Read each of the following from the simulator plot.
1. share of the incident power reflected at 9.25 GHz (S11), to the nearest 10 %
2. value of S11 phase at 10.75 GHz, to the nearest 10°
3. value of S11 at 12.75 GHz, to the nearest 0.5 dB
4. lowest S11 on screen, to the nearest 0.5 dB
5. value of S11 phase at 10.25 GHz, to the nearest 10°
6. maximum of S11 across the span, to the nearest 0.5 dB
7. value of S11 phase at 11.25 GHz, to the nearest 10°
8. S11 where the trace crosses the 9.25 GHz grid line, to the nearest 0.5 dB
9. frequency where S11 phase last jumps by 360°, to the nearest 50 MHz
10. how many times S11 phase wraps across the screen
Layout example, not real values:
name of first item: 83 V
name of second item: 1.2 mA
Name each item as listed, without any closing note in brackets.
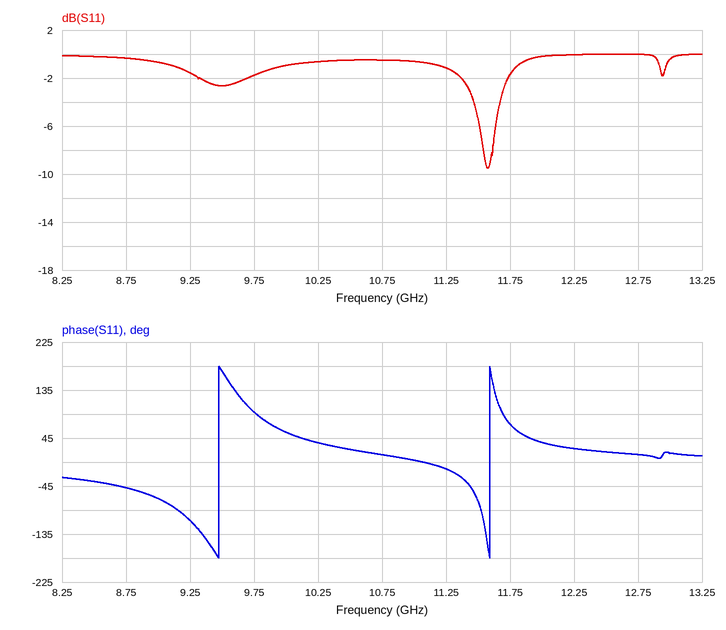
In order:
share of the incident power reflected at 9.25 GHz (S11), to the nearest 10 %: 70 %
value of S11 phase at 10.75 GHz, to the nearest 10°: 10°
value of S11 at 12.75 GHz, to the nearest 0.5 dB: 0.0 dB
lowest S11 on screen, to the nearest 0.5 dB: -9.5 dB
value of S11 phase at 10.25 GHz, to the nearest 10°: 40°
maximum of S11 across the span, to the nearest 0.5 dB: 0.0 dB
value of S11 phase at 11.25 GHz, to the nearest 10°: -10°
S11 where the trace crosses the 9.25 GHz grid line, to the nearest 0.5 dB: -1.5 dB
frequency where S11 phase last jumps by 360°, to the nearest 50 MHz: 11.60 GHz
how many times S11 phase wraps across the screen: 2
